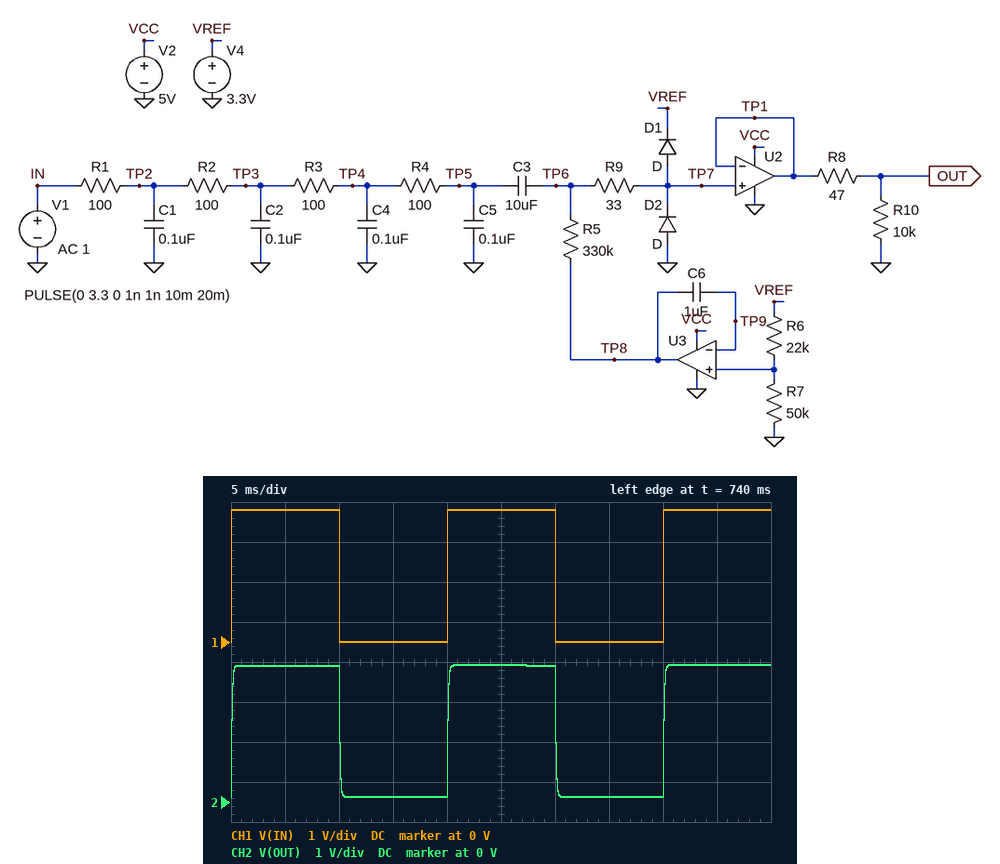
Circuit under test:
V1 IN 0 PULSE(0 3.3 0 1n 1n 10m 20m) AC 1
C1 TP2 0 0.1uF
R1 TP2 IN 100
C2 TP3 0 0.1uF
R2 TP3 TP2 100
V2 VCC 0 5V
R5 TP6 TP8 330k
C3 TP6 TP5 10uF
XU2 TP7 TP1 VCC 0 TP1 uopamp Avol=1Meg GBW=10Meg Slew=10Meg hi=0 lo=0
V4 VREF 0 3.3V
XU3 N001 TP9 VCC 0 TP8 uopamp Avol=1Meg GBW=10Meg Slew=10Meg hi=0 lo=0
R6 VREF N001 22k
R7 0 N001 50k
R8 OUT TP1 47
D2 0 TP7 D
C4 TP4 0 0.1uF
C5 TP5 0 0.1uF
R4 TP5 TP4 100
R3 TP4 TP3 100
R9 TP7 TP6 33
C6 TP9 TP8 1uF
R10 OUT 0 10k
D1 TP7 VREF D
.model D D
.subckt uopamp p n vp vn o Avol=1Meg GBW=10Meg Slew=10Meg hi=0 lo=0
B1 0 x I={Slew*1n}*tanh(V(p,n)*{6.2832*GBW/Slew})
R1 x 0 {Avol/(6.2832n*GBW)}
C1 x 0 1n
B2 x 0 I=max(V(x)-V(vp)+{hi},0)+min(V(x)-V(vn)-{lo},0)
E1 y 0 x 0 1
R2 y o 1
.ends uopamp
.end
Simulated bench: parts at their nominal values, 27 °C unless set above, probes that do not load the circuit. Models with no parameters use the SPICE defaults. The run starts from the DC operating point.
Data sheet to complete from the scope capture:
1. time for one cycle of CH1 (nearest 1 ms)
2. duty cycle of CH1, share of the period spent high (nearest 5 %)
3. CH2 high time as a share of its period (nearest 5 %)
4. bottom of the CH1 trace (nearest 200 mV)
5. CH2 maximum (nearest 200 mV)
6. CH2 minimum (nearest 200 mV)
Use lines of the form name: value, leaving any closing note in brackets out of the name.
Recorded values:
time for one cycle of CH1: 20 ms
duty cycle of CH1, share of the period spent high: 50 %
CH2 high time as a share of its period: 50 %
bottom of the CH1 trace: 0 V
CH2 maximum: 3.4 V
CH2 minimum: 200 mV
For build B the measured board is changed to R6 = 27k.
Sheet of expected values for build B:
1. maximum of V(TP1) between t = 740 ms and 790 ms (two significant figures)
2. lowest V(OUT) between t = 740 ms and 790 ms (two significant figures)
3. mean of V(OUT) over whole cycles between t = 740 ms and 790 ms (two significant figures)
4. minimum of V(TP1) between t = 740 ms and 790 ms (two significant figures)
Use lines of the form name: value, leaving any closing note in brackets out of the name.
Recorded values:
maximum of V(TP1) between t = 740 ms and 790 ms: 3.4 V
lowest V(OUT) between t = 740 ms and 790 ms: 98 mV
mean of V(OUT) over whole cycles between t = 740 ms and 790 ms: 1.7 V
minimum of V(TP1) between t = 740 ms and 790 ms: 99 mV
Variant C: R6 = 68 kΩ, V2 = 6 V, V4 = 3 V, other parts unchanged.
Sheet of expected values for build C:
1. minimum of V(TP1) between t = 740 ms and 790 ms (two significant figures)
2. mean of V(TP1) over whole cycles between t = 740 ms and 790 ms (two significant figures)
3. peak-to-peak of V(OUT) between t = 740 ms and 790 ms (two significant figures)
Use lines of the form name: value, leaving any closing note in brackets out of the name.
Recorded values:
minimum of V(TP1) between t = 740 ms and 790 ms: -4.5 mV
mean of V(TP1) over whole cycles between t = 740 ms and 790 ms: 1.6 V
peak-to-peak of V(OUT) between t = 740 ms and 790 ms: 3.2 V
